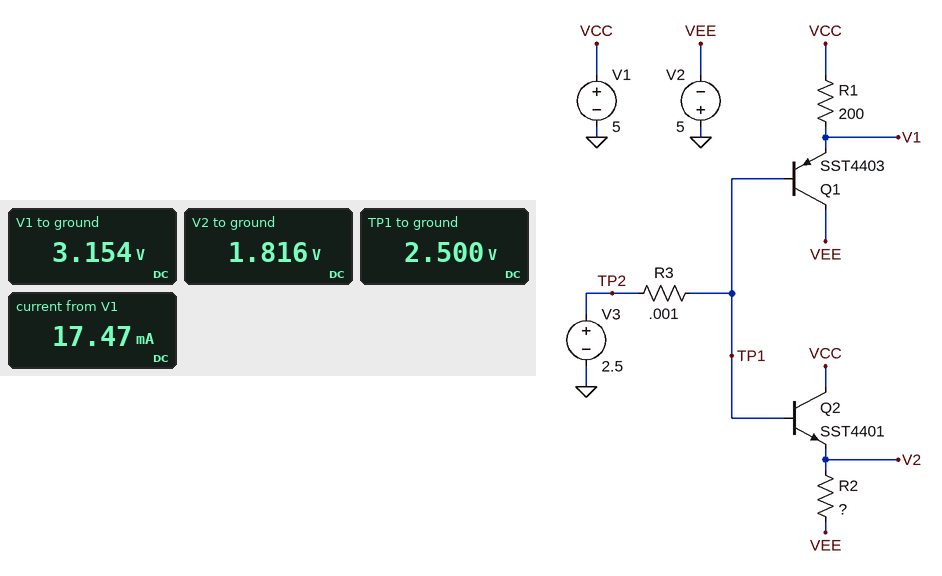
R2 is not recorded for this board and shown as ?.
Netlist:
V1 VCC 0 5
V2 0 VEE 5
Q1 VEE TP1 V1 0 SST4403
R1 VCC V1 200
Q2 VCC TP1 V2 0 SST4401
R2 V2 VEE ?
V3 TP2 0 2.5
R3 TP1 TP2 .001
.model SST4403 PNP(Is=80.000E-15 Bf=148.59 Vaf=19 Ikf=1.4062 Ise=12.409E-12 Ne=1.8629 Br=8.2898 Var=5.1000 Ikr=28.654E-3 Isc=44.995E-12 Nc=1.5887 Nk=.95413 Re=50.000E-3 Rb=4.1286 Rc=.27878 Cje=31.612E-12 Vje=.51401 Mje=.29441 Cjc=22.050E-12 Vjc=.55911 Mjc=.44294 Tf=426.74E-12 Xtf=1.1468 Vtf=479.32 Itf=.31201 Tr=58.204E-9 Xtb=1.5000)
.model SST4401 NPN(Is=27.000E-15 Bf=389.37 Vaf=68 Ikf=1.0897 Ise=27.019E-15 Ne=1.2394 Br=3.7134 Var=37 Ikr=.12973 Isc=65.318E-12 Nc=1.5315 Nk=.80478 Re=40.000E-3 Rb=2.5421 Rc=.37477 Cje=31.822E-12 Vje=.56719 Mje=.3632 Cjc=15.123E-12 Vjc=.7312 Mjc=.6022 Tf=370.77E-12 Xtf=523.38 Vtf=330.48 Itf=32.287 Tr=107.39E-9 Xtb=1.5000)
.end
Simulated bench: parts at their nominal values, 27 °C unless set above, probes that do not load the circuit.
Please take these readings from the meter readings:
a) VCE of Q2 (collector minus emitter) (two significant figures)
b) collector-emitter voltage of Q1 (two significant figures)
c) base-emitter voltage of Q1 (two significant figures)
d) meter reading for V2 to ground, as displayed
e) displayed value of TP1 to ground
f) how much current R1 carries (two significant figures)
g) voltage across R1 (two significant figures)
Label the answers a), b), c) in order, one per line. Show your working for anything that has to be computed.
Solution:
a) 5 V - 1.816 V = 3.2 V
b) -5 V - 3.154 V = -8.2 V
c) 2.5 V - 3.154 V = -650 mV
d) 1.816 V
e) 2.500 V
f) (5 V - 3.154 V) / 200 Ω = 9.2 mA
g) 5 V - 3.154 V = 1.8 V
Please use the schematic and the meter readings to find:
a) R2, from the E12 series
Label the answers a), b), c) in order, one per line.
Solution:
a) 820 Ω
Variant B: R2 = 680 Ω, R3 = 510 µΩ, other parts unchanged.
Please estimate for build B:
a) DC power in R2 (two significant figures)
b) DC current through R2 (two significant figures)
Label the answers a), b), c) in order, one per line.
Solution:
a) 68 mW
b) 10 mA
